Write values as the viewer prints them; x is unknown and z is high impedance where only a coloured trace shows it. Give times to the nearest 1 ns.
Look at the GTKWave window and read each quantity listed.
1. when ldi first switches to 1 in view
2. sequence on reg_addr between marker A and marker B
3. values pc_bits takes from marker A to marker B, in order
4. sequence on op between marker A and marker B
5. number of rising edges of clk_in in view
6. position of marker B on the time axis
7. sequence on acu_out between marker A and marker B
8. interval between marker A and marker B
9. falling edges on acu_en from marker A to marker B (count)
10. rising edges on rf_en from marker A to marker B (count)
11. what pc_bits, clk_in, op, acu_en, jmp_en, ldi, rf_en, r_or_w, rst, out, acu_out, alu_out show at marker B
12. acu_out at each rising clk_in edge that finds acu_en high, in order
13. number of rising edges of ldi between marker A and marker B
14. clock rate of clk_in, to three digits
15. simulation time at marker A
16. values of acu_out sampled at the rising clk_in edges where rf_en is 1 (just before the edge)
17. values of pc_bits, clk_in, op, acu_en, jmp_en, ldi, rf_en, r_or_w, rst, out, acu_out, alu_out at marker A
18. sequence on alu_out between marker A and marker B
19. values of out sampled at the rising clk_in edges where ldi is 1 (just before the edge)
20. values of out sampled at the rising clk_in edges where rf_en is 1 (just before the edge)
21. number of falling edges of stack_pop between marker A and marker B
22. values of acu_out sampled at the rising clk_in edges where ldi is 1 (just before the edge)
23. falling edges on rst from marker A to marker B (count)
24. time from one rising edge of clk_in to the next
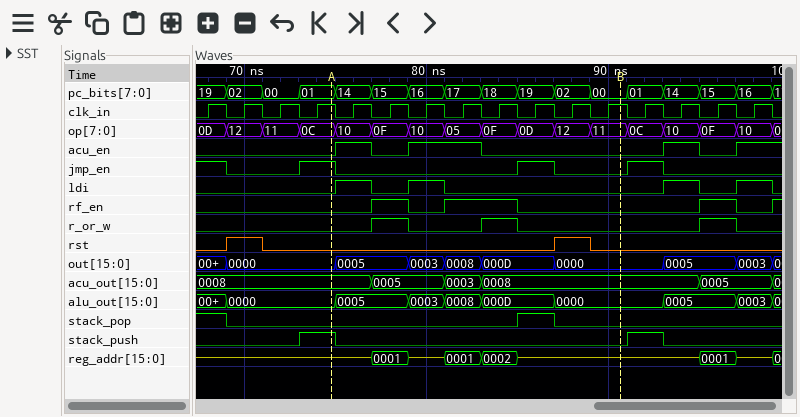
75 ns
z, 0001, z, 0001, 0002, z
01, 14, 15, 16, 17, 18, 19, 02, 00
0C, 10, 0F, 10, 05, 0F, 0D, 12, 11
16
91 ns
0008, 0005, 0003, 0008
16 ns
2
2
pc_bits=00, clk_in=1, op=11, acu_en=0, jmp_en=0, ldi=0, rf_en=0, r_or_w=0, rst=0, out=0000, acu_out=0008, alu_out=0000
0008, 0005, 0003, 0008, 0005
2
500 MHz
75 ns
0005, 0003, 0008, 0005
pc_bits=01, clk_in=1, op=0C, acu_en=0, jmp_en=1, ldi=0, rf_en=0, r_or_w=0, rst=0, out=0000, acu_out=0008, alu_out=0000
0000, 0005, 0003, 0008, 000D, 0000
0005, 0003, 0005, 0003
0005, 0008, 000D, 0005
1
0008, 0005, 0008, 0005
1
2 ns
